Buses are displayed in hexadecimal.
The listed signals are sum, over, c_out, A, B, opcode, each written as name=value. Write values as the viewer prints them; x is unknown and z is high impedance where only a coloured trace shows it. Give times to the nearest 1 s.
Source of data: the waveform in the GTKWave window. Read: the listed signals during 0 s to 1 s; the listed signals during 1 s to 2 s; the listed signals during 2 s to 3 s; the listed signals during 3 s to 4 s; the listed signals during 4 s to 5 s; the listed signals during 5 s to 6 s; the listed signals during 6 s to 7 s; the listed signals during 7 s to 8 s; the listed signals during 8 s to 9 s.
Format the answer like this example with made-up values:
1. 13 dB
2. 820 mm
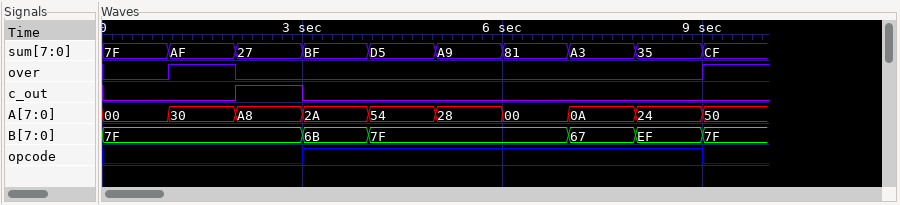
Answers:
1. sum=7F, over=0, c_out=0, A=00, B=7F, opcode=0
2. sum=AF, over=1, c_out=0, A=30, B=7F, opcode=0
3. sum=27, over=0, c_out=1, A=A8, B=7F, opcode=0
4. sum=BF, over=0, c_out=0, A=2A, B=6B, opcode=1
5. sum=D5, over=0, c_out=0, A=54, B=7F, opcode=1
6. sum=A9, over=0, c_out=0, A=28, B=7F, opcode=1
7. sum=81, over=0, c_out=0, A=00, B=7F, opcode=1
8. sum=A3, over=0, c_out=0, A=0A, B=67, opcode=1
9. sum=35, over=0, c_out=0, A=24, B=EF, opcode=1
